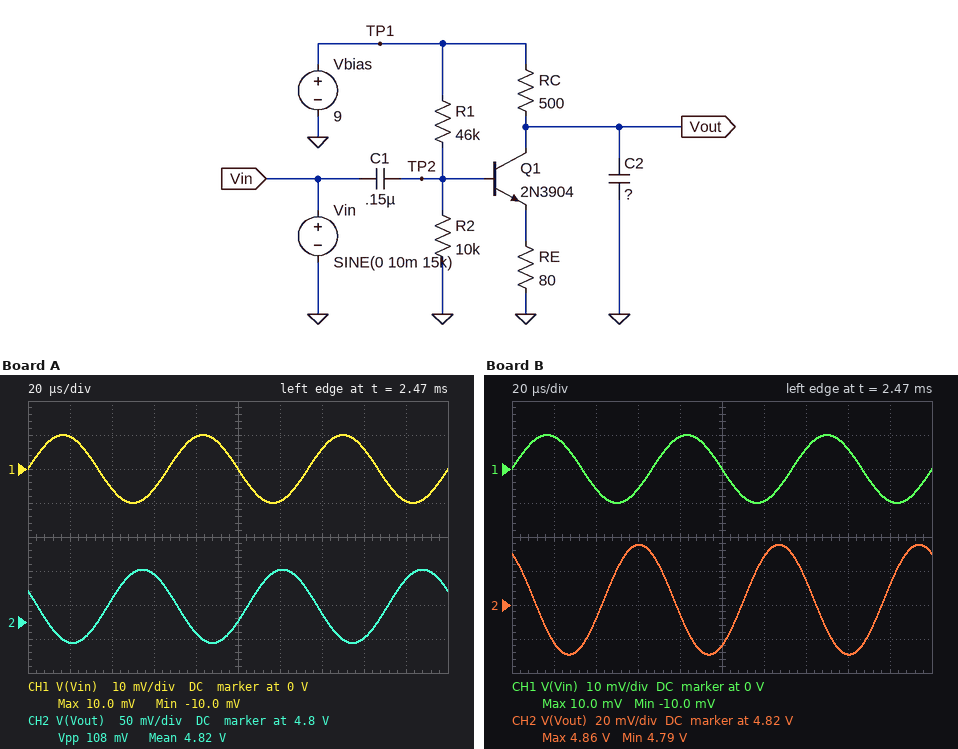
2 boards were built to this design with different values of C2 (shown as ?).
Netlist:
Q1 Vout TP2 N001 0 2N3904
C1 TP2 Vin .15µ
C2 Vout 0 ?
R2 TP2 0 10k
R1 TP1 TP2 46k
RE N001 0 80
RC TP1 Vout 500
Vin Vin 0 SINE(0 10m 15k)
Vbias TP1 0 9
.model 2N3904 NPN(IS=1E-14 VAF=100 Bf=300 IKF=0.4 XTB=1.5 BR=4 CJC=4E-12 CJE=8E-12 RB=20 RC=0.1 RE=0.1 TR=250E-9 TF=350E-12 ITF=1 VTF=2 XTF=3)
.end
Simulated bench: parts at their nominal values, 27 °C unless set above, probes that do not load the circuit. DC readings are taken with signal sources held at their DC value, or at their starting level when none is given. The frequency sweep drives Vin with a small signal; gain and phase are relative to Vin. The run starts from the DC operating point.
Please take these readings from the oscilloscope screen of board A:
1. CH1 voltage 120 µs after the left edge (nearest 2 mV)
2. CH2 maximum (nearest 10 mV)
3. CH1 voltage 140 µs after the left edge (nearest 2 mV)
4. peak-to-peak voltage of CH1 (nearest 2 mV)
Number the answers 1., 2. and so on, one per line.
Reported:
1. -10 mV
2. 4.88 V
3. 6 mV
4. 20 mV
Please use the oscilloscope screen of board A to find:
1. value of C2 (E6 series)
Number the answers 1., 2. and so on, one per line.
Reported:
1. 10 nF
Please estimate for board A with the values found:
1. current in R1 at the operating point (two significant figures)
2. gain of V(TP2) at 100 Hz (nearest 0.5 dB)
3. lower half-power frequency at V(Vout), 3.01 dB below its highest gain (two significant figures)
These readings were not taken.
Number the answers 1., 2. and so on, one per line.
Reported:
1. 170 µA
2. -6.0 dB
3. 170 Hz
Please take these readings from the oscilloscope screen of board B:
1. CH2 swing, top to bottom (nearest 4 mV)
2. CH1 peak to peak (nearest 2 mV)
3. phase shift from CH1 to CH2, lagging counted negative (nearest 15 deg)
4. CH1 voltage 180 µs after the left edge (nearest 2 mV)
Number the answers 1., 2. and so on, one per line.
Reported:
1. 64 mV
2. 20 mV
3. 120 deg
4. -10 mV
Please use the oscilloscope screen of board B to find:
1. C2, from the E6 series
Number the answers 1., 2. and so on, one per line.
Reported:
1. 33 nF
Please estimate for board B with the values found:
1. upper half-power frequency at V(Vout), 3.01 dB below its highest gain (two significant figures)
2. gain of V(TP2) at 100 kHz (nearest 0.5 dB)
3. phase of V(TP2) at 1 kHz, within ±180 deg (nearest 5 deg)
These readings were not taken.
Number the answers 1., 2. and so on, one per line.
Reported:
1. 10 kHz
2. 0 dB
3. 10 deg
